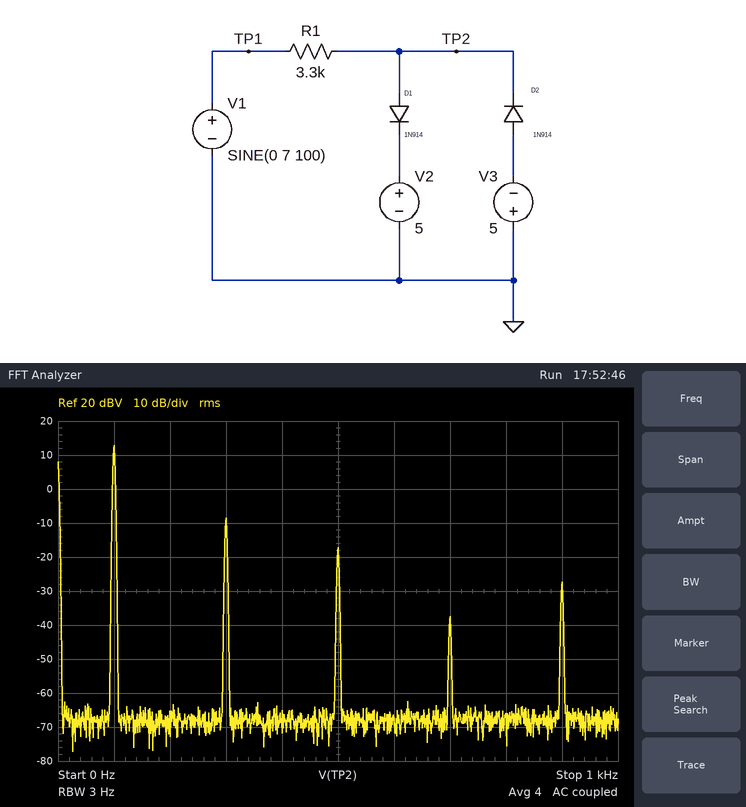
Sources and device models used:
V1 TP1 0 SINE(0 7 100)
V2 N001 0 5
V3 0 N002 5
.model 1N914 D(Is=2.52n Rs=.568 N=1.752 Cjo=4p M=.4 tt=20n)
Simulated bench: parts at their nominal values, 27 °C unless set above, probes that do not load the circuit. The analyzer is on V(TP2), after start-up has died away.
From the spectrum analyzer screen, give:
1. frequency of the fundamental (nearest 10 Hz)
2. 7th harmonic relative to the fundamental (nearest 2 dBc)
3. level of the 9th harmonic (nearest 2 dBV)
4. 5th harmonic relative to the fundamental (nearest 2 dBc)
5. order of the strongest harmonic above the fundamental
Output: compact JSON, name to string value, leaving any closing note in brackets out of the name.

{"frequency of the fundamental": "100 Hz", "7th harmonic relative to the fundamental": "-50 dBc", "level of the 9th harmonic": "-28 dBV", "5th harmonic relative to the fundamental": "-30 dBc", "order of the strongest harmonic above the fundamental": "3"}
